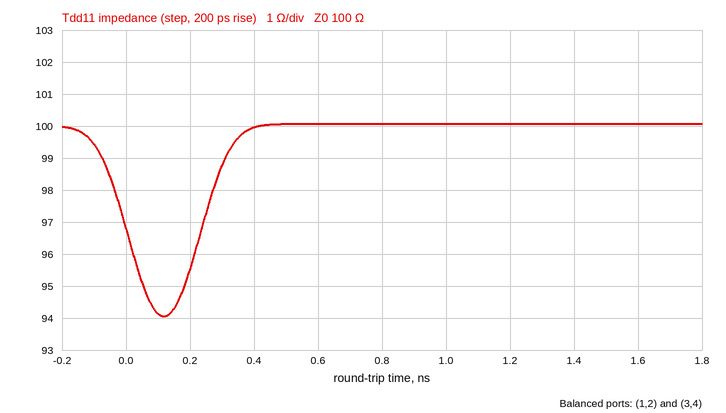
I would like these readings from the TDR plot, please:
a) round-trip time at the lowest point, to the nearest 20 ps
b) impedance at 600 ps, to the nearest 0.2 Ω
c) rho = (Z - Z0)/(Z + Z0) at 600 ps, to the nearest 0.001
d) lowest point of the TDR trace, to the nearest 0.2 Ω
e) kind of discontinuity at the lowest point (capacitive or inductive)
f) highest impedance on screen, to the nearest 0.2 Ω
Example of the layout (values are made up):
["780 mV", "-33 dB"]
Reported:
["120 ps", "100.0 Ω", "0.000", "94.0 Ω", "capacitive", "100.0 Ω"]
